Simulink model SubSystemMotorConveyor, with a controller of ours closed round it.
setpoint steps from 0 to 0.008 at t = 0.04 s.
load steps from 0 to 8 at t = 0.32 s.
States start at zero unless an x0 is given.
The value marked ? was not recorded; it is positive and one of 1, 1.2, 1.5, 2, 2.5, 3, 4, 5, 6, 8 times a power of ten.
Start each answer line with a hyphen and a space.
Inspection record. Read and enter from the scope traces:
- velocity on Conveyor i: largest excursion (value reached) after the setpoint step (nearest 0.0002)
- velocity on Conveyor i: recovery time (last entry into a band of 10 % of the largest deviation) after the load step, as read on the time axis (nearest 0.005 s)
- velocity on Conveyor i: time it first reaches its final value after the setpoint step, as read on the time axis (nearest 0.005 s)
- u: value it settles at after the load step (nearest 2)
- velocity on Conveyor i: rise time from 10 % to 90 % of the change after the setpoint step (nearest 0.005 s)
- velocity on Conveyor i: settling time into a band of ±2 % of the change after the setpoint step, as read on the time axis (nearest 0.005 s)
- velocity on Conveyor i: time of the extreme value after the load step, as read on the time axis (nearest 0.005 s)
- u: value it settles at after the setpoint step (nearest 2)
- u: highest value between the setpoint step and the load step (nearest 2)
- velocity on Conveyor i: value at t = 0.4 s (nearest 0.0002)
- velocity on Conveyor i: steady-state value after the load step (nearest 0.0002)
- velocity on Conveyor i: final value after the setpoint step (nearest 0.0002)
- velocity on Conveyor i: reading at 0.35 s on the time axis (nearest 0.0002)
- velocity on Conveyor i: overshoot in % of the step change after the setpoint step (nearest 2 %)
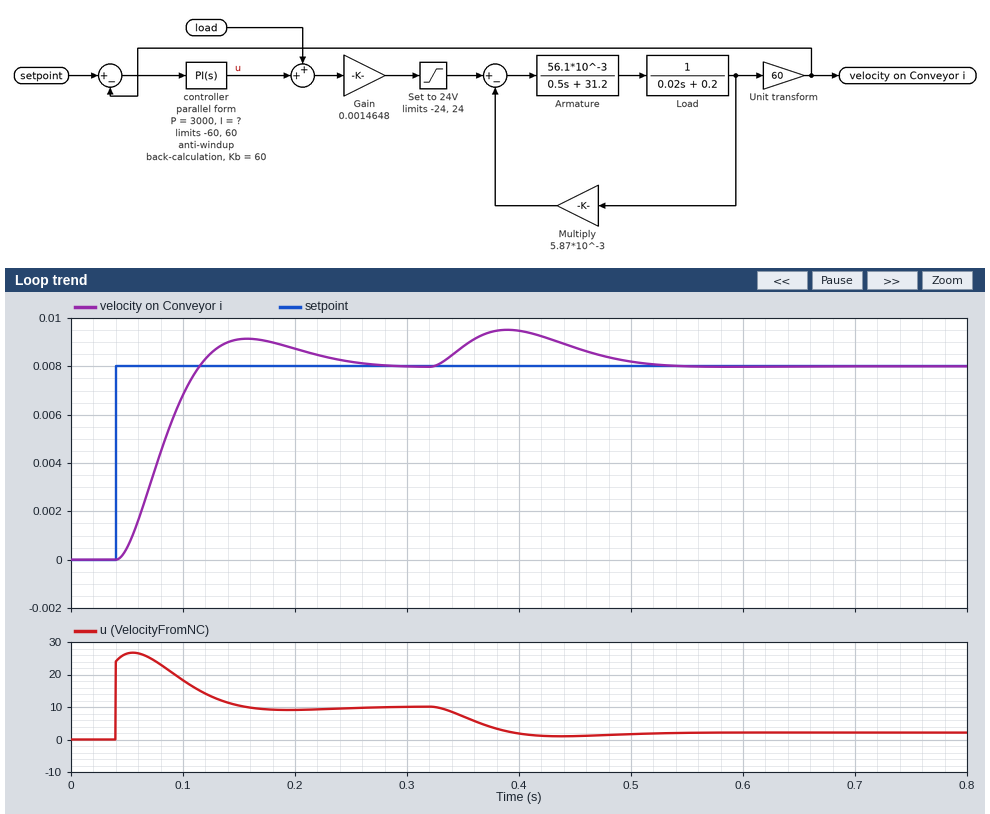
- 0.0092
- 0.505 s
- 0.115 s
- 2
- 0.050 s
- 0.255 s
- 0.390 s
- 10
- 26
- 0.0094
- 0.0080
- 0.0080
- 0.0088
- 14 %
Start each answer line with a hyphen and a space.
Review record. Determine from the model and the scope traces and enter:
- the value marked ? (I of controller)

- 50000
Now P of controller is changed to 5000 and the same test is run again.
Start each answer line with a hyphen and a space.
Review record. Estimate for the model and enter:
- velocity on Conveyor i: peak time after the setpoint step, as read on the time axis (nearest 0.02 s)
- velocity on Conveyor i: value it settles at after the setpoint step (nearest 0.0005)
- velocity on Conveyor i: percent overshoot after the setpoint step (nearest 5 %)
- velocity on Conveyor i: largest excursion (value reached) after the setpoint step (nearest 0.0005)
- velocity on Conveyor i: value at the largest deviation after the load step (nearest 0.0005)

- 0.12 s
- 0.0080
- 10 %
- 0.0085
- 0.0090
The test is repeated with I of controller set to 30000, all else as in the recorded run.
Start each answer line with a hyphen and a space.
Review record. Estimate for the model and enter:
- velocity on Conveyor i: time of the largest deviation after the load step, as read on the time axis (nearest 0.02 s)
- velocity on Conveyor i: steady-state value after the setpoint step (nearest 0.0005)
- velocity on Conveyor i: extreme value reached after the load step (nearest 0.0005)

- 0.40 s
- 0.0080
- 0.0095
